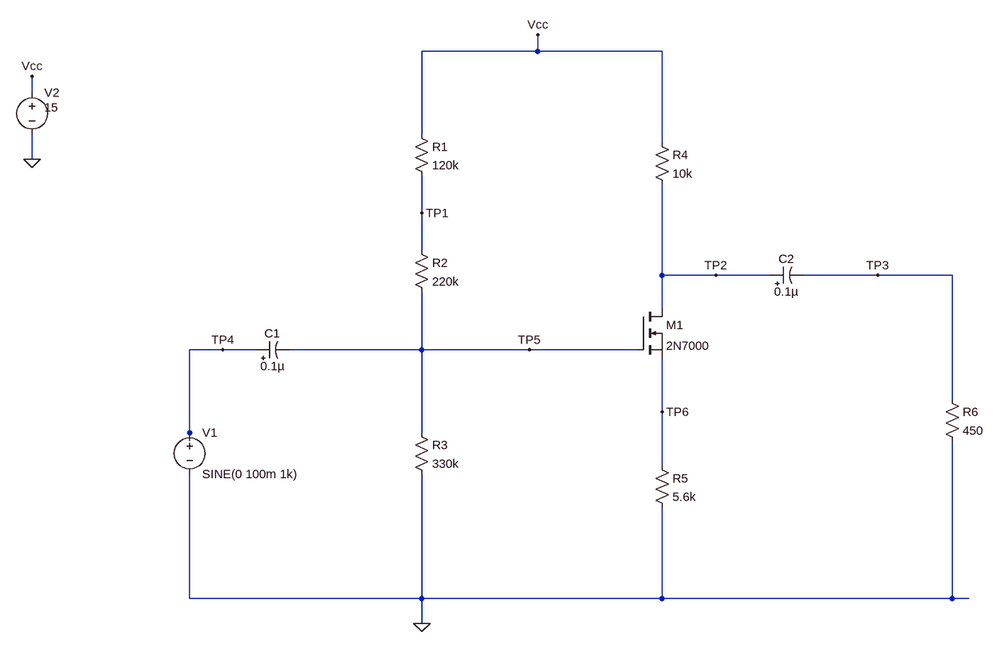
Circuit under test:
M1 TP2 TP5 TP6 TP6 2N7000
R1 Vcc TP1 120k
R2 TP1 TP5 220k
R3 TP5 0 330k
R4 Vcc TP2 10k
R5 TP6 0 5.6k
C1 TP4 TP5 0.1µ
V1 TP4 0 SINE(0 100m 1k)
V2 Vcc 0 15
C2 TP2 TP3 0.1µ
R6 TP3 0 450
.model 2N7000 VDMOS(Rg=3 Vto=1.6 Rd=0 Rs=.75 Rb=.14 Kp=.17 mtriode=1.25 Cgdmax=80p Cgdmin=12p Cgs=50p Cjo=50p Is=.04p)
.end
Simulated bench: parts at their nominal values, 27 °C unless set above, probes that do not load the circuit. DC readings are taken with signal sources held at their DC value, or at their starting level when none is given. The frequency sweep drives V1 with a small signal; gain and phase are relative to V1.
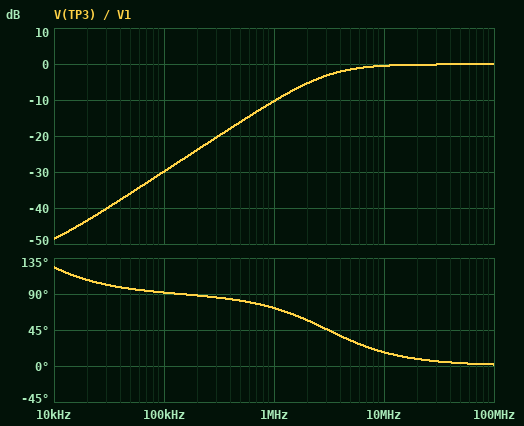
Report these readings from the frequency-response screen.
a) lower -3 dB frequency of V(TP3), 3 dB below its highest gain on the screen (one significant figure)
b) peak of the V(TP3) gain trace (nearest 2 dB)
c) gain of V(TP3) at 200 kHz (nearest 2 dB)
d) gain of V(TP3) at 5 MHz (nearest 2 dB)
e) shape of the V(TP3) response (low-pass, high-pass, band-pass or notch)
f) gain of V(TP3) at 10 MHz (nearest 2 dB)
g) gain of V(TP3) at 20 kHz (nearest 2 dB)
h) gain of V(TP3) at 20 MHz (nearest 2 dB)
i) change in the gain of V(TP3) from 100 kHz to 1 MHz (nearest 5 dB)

3 MHz
0 dB
-24 dB
-2 dB
high-pass
0 dB
-44 dB
0 dB
20 dB
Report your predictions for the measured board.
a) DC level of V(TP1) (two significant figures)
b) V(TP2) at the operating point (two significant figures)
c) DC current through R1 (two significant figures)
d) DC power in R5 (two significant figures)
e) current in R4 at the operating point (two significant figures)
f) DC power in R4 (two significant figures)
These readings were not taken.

12 V
5.4 V
22 µA
5.2 mW
960 µA
9.2 mW
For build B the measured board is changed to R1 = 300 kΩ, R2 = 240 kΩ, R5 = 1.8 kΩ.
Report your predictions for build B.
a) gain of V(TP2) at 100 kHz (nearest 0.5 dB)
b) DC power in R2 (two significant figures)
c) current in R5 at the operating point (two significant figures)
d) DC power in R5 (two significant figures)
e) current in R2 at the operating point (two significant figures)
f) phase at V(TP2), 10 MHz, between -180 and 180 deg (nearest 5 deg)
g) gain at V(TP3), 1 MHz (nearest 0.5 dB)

-31.0 dB
71 µW
1.3 mA
2.9 mW
17 µA
20 deg
-11.5 dB
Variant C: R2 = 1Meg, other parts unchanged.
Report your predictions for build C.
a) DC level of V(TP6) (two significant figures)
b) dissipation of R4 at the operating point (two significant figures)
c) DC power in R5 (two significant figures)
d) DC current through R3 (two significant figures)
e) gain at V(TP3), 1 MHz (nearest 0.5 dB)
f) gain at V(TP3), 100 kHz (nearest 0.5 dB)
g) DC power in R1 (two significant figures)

1.8 V
1.1 mW
600 µW
10 µA
-21.0 dB
-22.5 dB
13 µW
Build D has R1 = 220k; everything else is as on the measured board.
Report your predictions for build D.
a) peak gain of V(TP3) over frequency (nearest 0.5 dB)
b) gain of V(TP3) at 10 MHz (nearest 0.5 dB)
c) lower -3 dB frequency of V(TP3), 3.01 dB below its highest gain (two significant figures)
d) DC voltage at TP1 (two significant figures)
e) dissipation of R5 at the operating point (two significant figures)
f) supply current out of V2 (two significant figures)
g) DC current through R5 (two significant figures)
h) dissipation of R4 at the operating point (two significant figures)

0 dB
-1.0 dB
6.1 MHz
11 V
4.1 mW
870 µA
850 µA
7.3 mW
